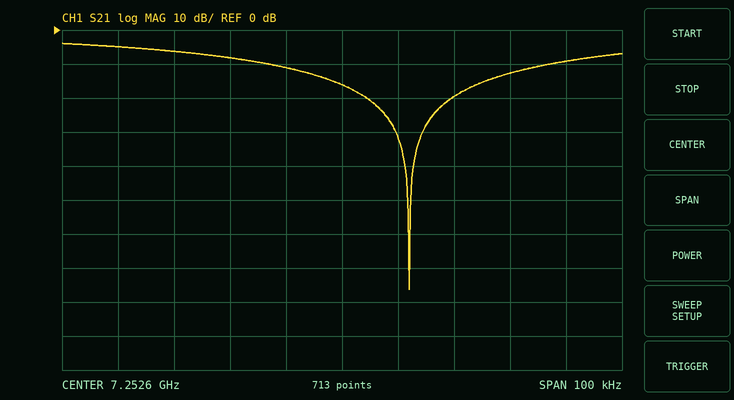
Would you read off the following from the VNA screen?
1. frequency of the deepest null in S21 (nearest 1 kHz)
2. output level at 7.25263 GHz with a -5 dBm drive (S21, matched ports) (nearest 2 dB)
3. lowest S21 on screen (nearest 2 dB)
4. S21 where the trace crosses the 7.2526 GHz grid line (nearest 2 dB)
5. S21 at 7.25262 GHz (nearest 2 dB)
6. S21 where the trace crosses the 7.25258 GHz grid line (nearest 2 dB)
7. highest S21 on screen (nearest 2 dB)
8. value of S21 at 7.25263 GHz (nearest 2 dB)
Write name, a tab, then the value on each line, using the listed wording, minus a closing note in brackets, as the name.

frequency of the deepest null in S21	7.252612 GHz
output level at 7.25263 GHz with a -5 dBm drive (S21, matched ports)	-18 dBm
lowest S21 on screen	-76 dB
S21 where the trace crosses the 7.2526 GHz grid line	-16 dB
S21 at 7.25262 GHz	-20 dB
S21 where the trace crosses the 7.25258 GHz grid line	-8 dB
highest S21 on screen	-4 dB
value of S21 at 7.25263 GHz	-12 dB
